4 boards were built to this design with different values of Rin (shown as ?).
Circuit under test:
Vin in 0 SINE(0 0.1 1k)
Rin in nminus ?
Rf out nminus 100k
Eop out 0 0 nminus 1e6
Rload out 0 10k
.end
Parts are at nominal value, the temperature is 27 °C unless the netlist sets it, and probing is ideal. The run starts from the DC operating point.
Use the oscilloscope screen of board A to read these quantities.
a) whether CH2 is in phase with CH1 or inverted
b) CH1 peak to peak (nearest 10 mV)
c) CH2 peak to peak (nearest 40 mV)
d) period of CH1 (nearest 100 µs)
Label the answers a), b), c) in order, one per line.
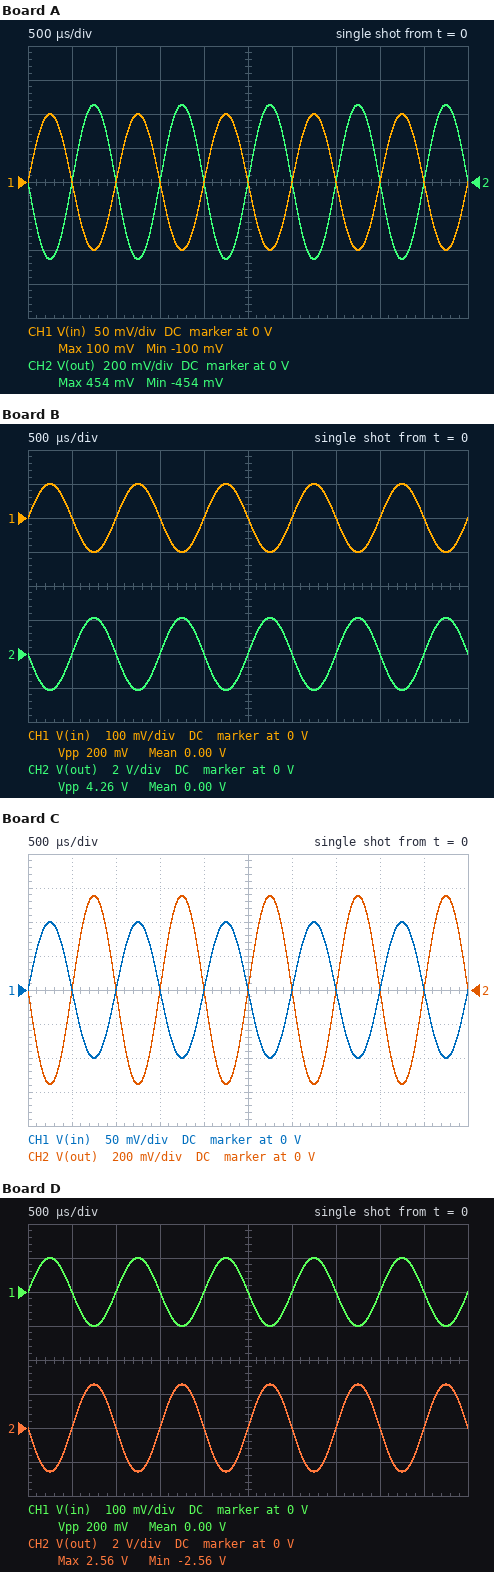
a) inverted
b) 200 mV
c) 920 mV
d) 1.0 ms
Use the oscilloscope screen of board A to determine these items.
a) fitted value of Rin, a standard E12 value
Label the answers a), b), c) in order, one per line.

a) 22 kΩ
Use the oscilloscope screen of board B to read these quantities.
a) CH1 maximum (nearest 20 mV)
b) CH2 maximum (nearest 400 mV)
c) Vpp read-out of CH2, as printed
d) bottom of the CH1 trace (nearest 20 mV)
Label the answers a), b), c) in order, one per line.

a) 100 mV
b) 2.0 V
c) 4.26 V
d) -100 mV
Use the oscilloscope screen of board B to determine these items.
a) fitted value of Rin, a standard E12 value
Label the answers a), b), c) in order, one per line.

a) 4.7 kΩ
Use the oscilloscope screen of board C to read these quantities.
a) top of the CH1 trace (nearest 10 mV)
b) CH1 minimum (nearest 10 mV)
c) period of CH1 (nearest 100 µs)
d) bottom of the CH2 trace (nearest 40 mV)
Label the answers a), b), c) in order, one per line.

a) 100 mV
b) -100 mV
c) 1.0 ms
d) -560 mV
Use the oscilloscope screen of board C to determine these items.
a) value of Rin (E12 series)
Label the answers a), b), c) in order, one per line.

a) 18 kΩ
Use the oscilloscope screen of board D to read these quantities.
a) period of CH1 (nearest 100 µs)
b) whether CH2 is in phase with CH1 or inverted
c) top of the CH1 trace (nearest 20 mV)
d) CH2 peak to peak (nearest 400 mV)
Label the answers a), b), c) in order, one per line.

a) 1.0 ms
b) inverted
c) 100 mV
d) 5.2 V
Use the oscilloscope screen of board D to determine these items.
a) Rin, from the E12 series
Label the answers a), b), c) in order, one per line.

a) 3.9 kΩ
